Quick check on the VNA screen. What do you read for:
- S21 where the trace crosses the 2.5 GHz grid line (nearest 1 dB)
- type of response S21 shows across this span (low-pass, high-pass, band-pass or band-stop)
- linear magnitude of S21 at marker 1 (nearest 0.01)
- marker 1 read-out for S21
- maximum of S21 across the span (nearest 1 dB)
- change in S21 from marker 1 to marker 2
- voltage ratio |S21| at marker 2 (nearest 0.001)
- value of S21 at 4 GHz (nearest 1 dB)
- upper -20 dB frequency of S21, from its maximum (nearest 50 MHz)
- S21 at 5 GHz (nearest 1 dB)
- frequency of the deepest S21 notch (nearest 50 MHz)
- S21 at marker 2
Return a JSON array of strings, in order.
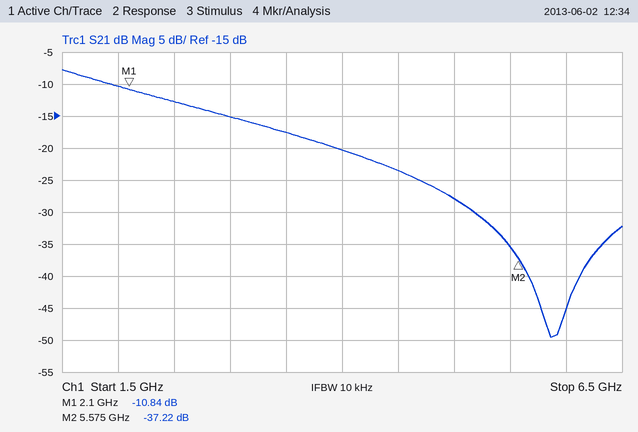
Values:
["-13 dB", "low-pass", "0.29", "-10.84 dB", "-8 dB", "-26.38 dB", "0.014", "-20 dB", "5.00 GHz", "-28 dB", "5.85 GHz", "-37.22 dB"]
